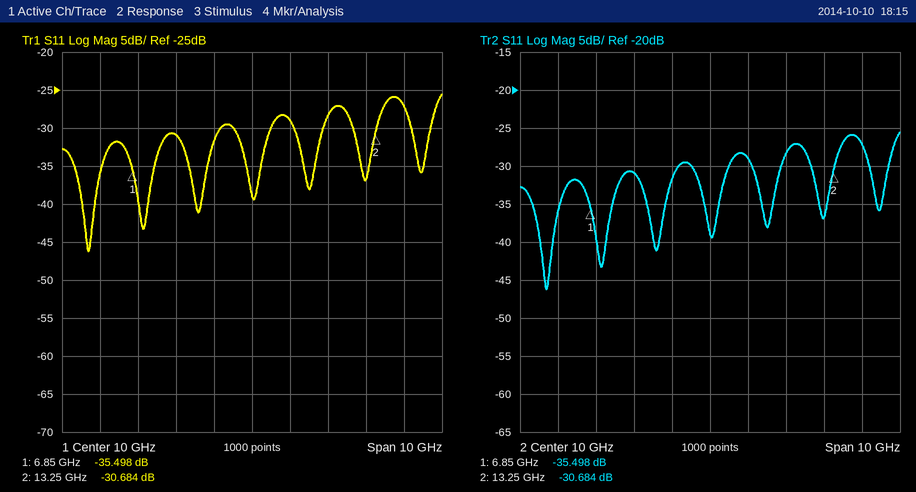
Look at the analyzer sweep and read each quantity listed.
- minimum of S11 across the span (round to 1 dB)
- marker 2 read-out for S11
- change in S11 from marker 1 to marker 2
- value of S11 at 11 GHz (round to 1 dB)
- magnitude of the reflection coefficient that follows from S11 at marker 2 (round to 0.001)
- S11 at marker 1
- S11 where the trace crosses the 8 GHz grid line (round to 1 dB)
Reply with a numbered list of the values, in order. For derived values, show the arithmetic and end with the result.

1. -46 dB
2. -30.684 dB
3. -30.684 − (-35.498) = 4.814 dB
4. -29 dB
5. 10^(-30.684/20) ≈ 0.029
6. -35.498 dB
7. -31 dB
